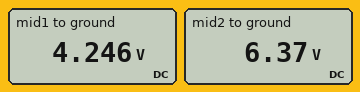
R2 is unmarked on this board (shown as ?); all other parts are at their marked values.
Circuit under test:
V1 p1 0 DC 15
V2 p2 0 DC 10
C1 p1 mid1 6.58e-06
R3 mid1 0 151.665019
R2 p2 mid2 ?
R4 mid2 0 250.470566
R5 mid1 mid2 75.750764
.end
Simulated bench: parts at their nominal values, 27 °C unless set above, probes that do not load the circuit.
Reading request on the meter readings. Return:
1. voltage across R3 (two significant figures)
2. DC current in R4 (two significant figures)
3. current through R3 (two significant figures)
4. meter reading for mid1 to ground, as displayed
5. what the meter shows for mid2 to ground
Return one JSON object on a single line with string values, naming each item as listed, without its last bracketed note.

{"voltage across R3": "4.2 V", "DC current in R4": "25 mA", "current through R3": "28 mA", "meter reading for mid1 to ground, as displayed": "4.246 V", "what the meter shows for mid2 to ground": "6.37 V"}
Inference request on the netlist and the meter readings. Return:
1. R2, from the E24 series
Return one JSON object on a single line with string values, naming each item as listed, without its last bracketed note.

{"R2, from the E24 series": "68 Ω"}
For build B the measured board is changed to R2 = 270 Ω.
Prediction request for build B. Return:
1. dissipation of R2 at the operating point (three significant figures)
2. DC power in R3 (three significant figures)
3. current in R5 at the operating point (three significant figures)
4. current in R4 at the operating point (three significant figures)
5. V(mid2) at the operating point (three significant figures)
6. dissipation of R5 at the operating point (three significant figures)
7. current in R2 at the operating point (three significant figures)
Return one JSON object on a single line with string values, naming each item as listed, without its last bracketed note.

{"dissipation of R2 at the operating point": "178 mW", "DC power in R3": "27.5 mW", "current in R5 at the operating point": "13.5 mA", "current in R4 at the operating point": "12.2 mA", "V(mid2) at the operating point": "3.06 V", "dissipation of R5 at the operating point": "13.7 mW", "current in R2 at the operating point": "25.7 mA"}
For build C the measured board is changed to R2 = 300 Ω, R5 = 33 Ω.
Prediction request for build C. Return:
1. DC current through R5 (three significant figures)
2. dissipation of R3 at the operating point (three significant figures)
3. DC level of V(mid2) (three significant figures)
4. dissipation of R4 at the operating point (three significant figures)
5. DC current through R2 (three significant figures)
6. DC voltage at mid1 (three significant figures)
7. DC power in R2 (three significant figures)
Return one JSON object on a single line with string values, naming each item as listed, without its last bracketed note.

{"DC current through R5": "14.2 mA", "dissipation of R3 at the operating point": "30.4 mW", "DC level of V(mid2)": "2.62 V", "dissipation of R4 at the operating point": "27.3 mW", "DC current through R2": "24.6 mA", "DC voltage at mid1": "2.15 V", "DC power in R2": "182 mW"}
